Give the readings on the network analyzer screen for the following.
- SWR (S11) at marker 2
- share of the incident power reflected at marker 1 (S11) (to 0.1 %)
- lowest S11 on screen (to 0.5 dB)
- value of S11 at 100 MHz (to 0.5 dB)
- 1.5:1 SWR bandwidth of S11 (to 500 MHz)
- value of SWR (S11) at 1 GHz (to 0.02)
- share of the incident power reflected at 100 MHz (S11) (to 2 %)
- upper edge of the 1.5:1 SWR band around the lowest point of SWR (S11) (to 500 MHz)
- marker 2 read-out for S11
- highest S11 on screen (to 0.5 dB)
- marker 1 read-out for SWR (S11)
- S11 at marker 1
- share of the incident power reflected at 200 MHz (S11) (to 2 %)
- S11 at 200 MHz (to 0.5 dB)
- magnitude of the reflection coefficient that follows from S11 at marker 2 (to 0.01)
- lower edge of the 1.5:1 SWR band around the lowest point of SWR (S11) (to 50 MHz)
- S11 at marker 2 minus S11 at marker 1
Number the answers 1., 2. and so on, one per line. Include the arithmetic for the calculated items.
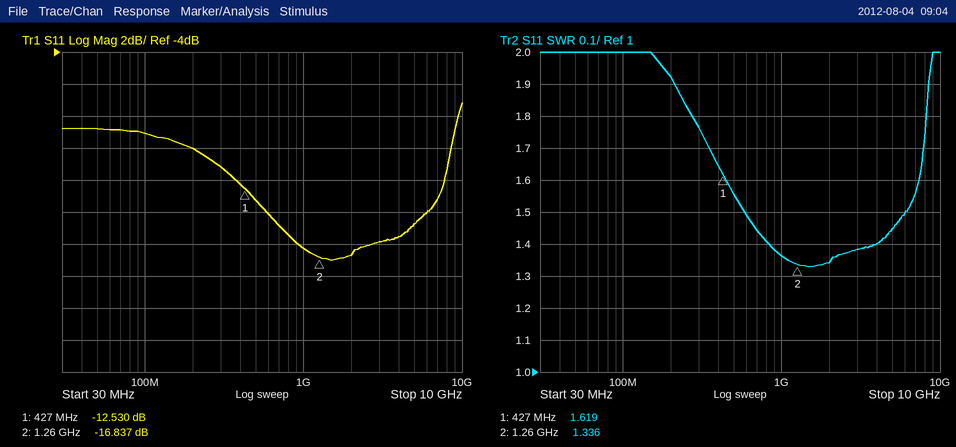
1. 1.336
2. 10^(-12.53/10) ≈ 5.6 %
3. -17.0 dB
4. -9.0 dB
5. 6.0 GHz − 600 MHz = 5.40 GHz
6. 1.36
7. 10^(-9/10) ≈ 12.6 %, so 12 % to the nearest 2 %
8. 6.0 GHz
9. -16.837 dB
10. -7.0 dB
11. 1.619
12. -12.530 dB
13. 10^(-10/10) ≈ 10 %
14. -10.0 dB
15. 10^(-16.837/20) ≈ 0.14
16. 600 MHz
17. -16.837 − (-12.53) = -4.307 dB
